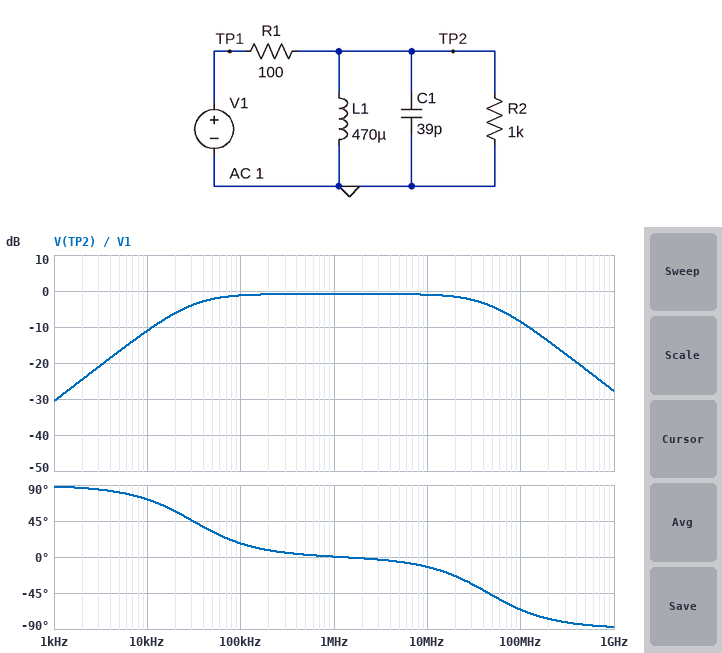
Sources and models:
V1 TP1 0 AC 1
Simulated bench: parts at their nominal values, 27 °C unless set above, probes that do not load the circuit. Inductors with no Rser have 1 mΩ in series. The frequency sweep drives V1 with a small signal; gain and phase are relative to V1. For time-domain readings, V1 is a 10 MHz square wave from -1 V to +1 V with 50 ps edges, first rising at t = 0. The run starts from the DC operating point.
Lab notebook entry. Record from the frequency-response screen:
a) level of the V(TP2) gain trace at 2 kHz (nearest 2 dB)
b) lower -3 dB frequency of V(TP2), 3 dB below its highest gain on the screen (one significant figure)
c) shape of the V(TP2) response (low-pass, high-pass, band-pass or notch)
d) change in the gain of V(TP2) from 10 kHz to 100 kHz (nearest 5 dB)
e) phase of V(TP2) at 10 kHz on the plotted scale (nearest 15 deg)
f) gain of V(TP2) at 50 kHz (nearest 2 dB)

-24 dB
30 kHz
band-pass
10 dB
75 deg
-2 dB
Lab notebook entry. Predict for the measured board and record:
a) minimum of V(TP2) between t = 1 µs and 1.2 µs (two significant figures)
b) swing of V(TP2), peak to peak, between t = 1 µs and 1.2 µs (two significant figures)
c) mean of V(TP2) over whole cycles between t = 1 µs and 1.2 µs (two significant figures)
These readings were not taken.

-190 mV
1.8 V
740 mV
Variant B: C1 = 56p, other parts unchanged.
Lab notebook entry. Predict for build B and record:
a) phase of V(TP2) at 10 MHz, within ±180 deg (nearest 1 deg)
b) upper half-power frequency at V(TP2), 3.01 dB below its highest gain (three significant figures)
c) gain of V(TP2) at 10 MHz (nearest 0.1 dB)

-18 deg
31.3 MHz
-1.2 dB
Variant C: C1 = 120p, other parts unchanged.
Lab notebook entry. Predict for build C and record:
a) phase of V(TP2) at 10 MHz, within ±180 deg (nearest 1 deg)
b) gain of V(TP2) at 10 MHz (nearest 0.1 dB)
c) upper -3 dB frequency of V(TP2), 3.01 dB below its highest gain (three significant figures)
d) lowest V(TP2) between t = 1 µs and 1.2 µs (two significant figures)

-34 deg
-2.5 dB
14.6 MHz
-170 mV
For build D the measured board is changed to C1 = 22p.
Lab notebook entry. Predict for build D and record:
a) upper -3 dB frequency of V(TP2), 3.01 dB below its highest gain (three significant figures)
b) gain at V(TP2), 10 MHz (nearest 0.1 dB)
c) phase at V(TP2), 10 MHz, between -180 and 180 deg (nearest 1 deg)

79.6 MHz
-0.9 dB
-7 deg
